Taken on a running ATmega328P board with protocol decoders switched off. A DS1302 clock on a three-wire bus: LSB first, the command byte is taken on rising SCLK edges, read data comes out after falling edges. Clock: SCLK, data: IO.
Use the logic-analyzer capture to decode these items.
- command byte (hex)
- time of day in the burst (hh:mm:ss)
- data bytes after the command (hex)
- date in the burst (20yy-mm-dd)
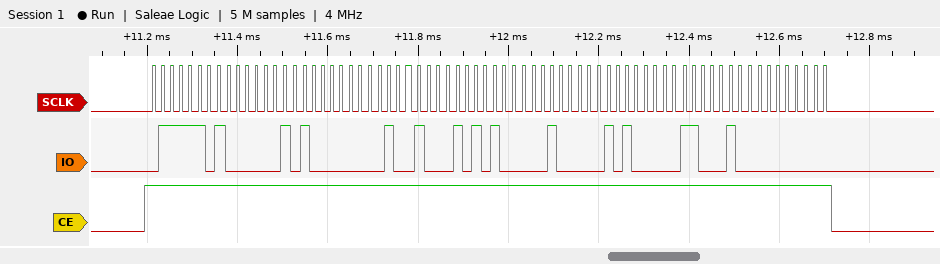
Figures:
0xBE
12:01:40
40 01 12 15 04 05 23 00
2023-04-15
